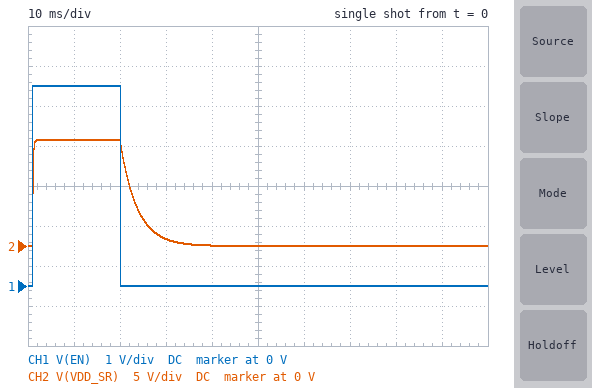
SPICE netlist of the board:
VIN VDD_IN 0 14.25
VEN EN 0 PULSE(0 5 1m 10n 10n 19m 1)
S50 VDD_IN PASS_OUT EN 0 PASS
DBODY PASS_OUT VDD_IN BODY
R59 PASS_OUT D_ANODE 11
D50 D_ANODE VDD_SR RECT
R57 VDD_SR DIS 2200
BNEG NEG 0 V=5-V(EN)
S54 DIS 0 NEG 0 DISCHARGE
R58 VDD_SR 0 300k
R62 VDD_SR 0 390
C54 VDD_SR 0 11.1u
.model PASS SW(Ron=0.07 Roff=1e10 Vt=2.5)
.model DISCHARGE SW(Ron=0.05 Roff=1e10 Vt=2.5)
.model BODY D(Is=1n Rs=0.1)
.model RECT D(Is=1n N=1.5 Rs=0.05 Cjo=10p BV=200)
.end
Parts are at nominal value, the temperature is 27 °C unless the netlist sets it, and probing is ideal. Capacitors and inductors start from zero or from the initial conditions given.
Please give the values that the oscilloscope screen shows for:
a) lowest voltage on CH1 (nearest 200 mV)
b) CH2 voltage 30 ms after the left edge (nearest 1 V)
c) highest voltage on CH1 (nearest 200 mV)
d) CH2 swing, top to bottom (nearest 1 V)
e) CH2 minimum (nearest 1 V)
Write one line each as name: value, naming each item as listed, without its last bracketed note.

lowest voltage on CH1: 0 V
CH2 voltage 30 ms after the left edge: 1 V
highest voltage on CH1: 5.0 V
CH2 swing, top to bottom: 13 V
CH2 minimum: 0 V
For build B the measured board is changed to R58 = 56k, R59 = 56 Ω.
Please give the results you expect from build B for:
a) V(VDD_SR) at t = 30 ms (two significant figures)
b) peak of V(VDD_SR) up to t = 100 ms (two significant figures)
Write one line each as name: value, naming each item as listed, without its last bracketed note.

V(VDD_SR) at t = 30 ms: 770 mV
peak of V(VDD_SR) up to t = 100 ms: 12 V
